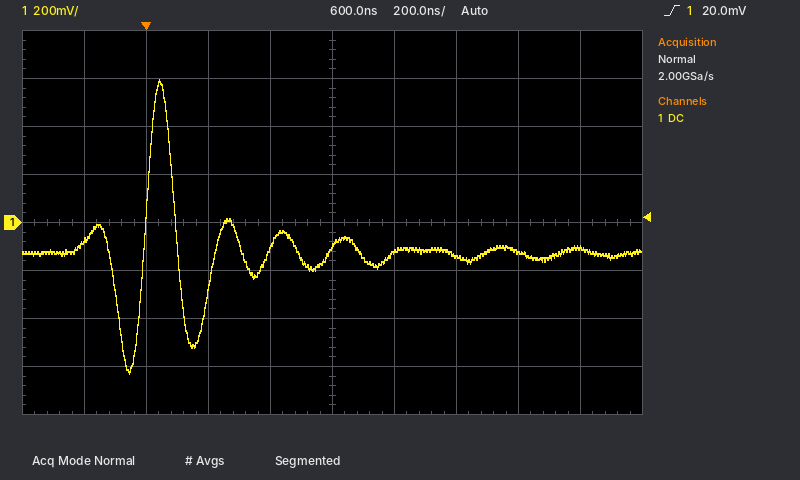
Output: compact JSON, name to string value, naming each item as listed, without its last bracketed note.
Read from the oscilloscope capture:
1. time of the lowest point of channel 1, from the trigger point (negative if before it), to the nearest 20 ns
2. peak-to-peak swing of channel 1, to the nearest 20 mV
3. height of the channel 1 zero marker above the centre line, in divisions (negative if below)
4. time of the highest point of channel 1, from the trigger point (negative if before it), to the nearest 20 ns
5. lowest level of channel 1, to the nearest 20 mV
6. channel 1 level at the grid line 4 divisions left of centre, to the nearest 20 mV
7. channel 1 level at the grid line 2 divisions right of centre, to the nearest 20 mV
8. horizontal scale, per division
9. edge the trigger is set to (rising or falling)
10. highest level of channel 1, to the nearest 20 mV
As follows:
{"time of the lowest point of channel 1, from the trigger point (negative if before it), to the nearest 20 ns": "-60 ns", "peak-to-peak swing of channel 1, to the nearest 20 mV": "1.22 V", "height of the channel 1 zero marker above the centre line, in divisions": "0.0 div", "time of the highest point of channel 1, from the trigger point (negative if before it), to the nearest 20 ns": "+40 ns", "lowest level of channel 1, to the nearest 20 mV": "-620 mV", "channel 1 level at the grid line 4 divisions left of centre, to the nearest 20 mV": "-80 mV", "channel 1 level at the grid line 2 divisions right of centre, to the nearest 20 mV": "-140 mV", "horizontal scale, per division": "200 ns", "edge the trigger is set to": "rising", "highest level of channel 1, to the nearest 20 mV": "600 mV"}
